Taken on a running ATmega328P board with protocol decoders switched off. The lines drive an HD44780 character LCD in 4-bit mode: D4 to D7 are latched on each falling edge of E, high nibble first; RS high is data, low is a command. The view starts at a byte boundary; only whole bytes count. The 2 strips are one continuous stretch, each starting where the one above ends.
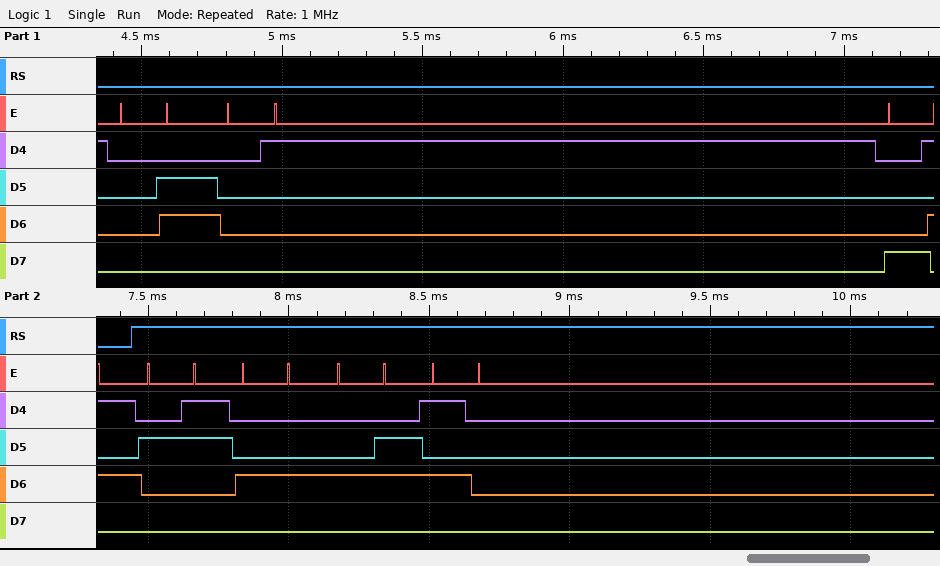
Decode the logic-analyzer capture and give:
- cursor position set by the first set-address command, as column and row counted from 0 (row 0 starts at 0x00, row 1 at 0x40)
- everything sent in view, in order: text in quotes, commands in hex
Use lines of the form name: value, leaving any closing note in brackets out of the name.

cursor position set by the first set-address command, as column and row counted from 0: column 5, row 0
everything sent in view, in order: text in quotes, commands in hex: 0x06 0x01 0x85 "#DFP"
